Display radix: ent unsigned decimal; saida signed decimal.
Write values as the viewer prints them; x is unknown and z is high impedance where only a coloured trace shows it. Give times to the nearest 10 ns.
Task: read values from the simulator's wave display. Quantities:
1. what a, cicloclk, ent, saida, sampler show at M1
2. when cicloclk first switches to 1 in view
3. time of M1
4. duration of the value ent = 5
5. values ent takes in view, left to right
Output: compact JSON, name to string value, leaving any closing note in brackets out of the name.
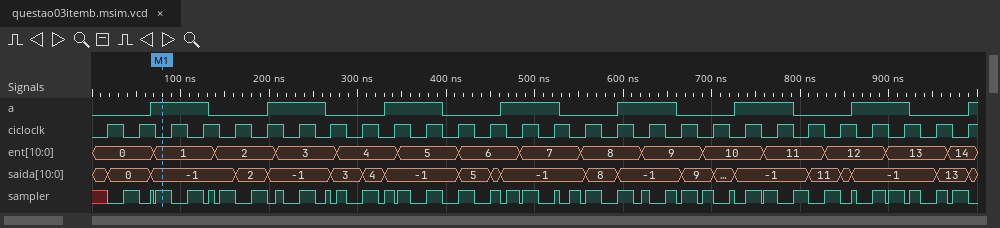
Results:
{"what a, cicloclk, ent, saida, sampler show at M1": "a=1, cicloclk=0, ent=1, saida=-1, sampler=1", "when cicloclk first switches to 1 in view": "20 ns", "time of M1": "80 ns", "duration of the value ent = 5": "70 ns", "values ent takes in view, left to right": "0, 1, 2, 3, 4, 5, 6, 7, 8, 9, 10, 11, 12, 13, 14"}
